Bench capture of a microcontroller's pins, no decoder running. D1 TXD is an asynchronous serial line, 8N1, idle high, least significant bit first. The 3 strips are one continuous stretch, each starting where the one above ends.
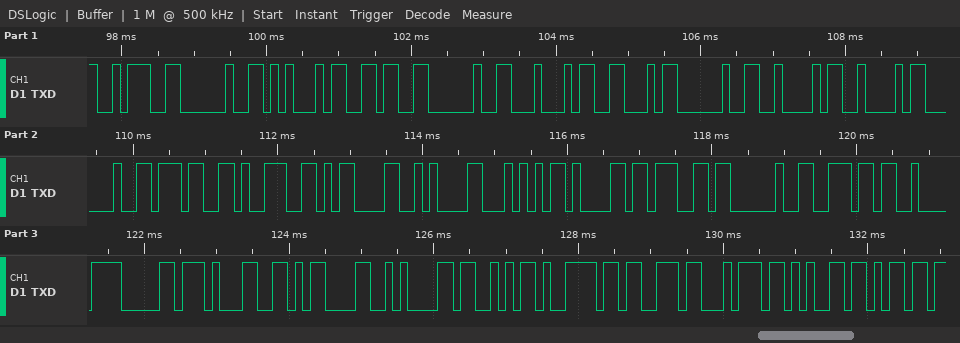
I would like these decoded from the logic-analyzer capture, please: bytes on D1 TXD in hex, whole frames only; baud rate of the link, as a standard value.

3A 20 45 36 20 44 46 20 42 42 20 37 39 0D 0A 54 61 67 20 6E C2 B0 31 0D 0A 53 79 73 74 65 6D
9600 baud
